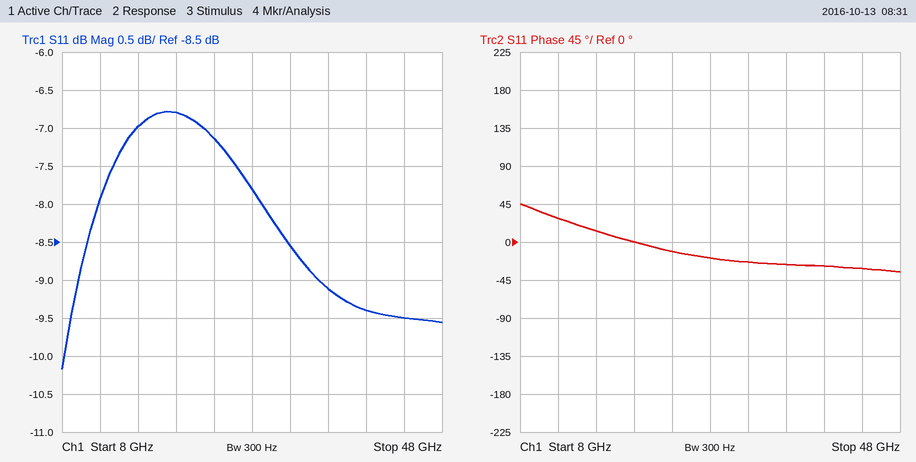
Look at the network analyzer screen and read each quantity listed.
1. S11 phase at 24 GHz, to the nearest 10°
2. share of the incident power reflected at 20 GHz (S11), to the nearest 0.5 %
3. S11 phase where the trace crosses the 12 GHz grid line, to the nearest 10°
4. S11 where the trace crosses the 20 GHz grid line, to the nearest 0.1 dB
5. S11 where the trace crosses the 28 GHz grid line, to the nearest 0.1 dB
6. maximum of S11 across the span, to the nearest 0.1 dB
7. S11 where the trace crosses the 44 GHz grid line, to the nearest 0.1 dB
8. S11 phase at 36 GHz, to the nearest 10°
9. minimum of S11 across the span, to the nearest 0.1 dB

-10°
21.0 %
30°
-6.8 dB
-7.8 dB
-6.8 dB
-9.5 dB
-30°
-10.2 dB
